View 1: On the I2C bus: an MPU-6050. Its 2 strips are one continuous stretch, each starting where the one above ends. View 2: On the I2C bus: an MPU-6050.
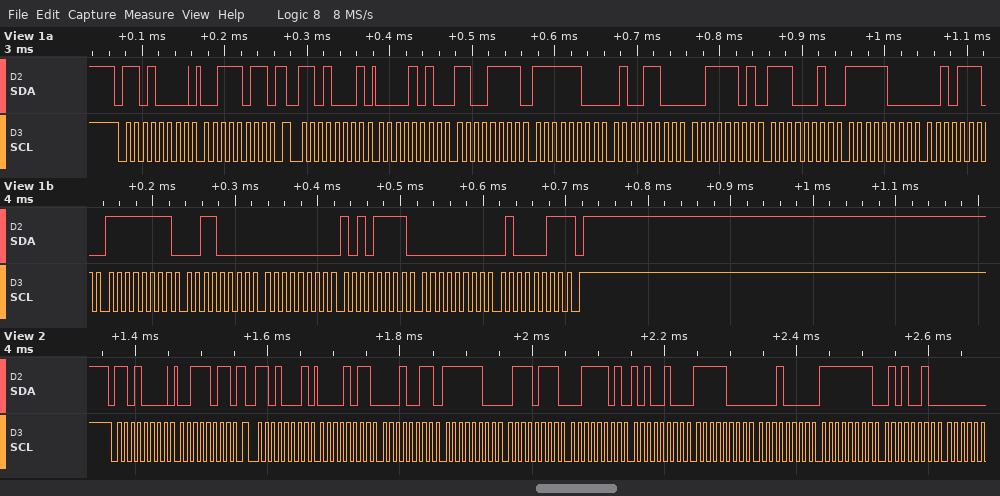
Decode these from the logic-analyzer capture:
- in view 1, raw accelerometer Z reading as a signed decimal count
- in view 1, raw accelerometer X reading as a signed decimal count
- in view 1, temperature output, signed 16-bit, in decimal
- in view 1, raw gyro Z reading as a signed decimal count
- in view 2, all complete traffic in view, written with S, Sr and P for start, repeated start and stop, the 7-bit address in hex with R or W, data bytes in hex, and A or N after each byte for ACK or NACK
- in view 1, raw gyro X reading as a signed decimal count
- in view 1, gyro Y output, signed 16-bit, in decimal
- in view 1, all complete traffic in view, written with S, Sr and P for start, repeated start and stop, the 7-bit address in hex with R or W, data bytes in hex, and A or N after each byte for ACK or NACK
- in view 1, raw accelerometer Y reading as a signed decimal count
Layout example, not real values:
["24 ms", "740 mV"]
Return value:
["15842", "2767", "-2002", "67", "S 68W A 3B A Sr 68R A 0B A 13 A FC A 77 A 3D A A4 A F8 A 10 A FF A 52 A", "-208", "175", "S 68W A 3B A Sr 68R A 0A A CF A FC A 4C A 3D A E2 A F8 A 2E A FF A 30 A 00 A AF A 00 A 43 N P", "-948"]
